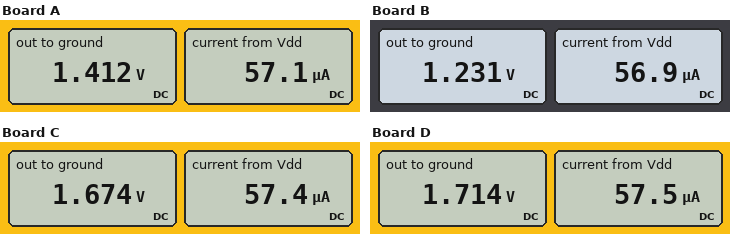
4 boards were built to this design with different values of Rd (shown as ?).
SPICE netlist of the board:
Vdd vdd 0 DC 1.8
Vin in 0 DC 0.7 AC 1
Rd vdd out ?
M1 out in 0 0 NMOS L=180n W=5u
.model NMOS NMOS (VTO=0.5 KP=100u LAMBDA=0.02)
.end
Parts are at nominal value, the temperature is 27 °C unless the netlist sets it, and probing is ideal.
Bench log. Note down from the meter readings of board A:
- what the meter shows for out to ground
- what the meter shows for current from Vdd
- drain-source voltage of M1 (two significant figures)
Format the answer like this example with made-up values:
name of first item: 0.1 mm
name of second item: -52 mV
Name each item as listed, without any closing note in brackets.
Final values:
what the meter shows for out to ground: 1.412 V
what the meter shows for current from Vdd: 57.1 µA
drain-source voltage of M1: 1.4 V
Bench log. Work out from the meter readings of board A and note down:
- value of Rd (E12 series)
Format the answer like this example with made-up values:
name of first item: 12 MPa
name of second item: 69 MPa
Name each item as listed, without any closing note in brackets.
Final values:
value of Rd: 6.8 kΩ
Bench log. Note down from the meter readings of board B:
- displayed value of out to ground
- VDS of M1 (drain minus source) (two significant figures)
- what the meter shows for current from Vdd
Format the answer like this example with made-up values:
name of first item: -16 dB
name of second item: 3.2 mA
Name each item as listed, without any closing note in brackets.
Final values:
displayed value of out to ground: 1.231 V
VDS of M1 (drain minus source): 1.2 V
what the meter shows for current from Vdd: 56.9 µA
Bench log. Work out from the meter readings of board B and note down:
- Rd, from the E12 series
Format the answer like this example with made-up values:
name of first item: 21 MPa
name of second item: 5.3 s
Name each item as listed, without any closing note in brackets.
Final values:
Rd, from the E12 series: 10 kΩ
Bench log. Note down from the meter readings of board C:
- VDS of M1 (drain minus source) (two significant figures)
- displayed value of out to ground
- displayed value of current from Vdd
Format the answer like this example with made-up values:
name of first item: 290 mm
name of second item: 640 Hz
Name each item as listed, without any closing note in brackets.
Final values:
VDS of M1 (drain minus source): 1.7 V
displayed value of out to ground: 1.674 V
displayed value of current from Vdd: 57.4 µA
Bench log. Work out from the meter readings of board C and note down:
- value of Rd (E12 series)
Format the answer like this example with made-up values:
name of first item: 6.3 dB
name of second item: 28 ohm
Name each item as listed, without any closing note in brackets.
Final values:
value of Rd: 2.2 kΩ
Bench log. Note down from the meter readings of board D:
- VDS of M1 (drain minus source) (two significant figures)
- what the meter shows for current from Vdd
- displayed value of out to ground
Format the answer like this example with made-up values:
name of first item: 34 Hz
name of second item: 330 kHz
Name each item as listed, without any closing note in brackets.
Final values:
VDS of M1 (drain minus source): 1.7 V
what the meter shows for current from Vdd: 57.5 µA
displayed value of out to ground: 1.714 V
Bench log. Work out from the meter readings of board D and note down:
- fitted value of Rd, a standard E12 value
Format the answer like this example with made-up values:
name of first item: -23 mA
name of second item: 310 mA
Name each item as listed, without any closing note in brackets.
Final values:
fitted value of Rd, a standard E12 value: 1.5 kΩ
